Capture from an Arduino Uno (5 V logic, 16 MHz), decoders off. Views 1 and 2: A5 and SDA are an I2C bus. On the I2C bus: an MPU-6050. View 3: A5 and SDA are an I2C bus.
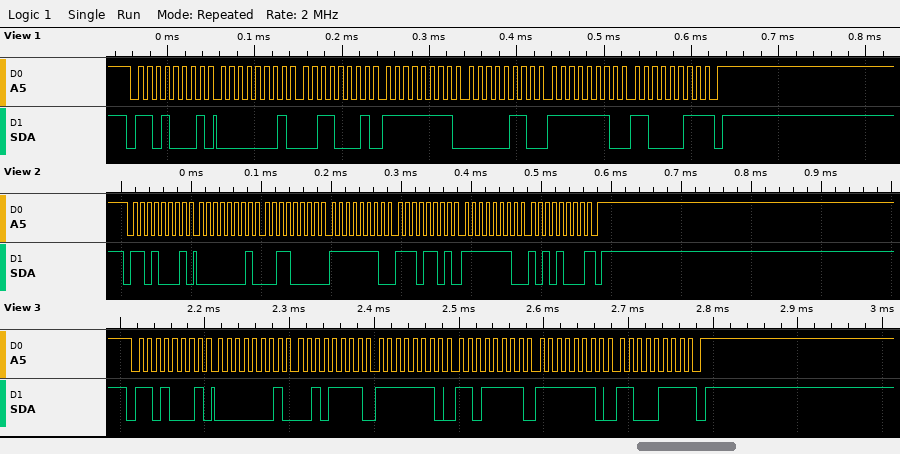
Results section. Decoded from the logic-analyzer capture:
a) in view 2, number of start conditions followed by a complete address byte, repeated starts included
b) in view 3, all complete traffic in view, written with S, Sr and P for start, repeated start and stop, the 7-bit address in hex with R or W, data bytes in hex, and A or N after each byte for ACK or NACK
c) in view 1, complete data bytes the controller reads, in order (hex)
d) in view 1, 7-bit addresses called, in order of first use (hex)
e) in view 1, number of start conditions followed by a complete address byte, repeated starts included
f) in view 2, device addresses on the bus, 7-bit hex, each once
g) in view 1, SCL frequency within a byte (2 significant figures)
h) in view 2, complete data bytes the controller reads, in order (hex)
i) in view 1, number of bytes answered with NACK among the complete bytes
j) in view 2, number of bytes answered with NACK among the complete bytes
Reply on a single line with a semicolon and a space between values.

1; S 68R A 01 A 2F A FE A DF A FE A C7 N P; 01 31 FF 06 FE C3; 0x68; 1; 0x68; 100 kHz; 01 30 FE ED FE A8; 1; 1
